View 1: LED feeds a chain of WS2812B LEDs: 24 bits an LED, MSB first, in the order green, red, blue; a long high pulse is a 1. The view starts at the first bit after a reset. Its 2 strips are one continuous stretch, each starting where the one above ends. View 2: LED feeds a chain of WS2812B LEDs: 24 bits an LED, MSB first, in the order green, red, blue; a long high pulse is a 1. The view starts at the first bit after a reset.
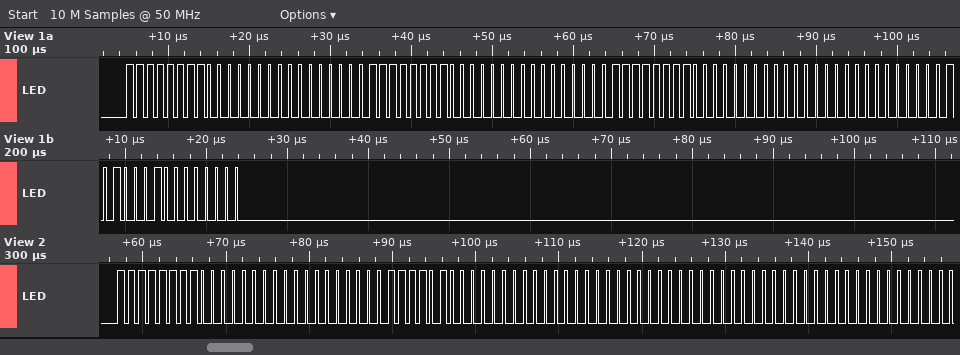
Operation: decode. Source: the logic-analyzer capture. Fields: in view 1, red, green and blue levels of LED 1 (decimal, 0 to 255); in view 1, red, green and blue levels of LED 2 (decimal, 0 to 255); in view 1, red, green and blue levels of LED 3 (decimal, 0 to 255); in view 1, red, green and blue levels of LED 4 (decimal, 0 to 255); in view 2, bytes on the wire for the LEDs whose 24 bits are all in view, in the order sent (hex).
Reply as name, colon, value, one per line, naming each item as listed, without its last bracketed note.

in view 1, red, green and blue levels of LED 1: 0, 255, 0
in view 1, red, green and blue levels of LED 2: 0, 255, 0
in view 1, red, green and blue levels of LED 3: 0, 255, 0
in view 1, red, green and blue levels of LED 4: 81, 0, 0
in view 2, bytes on the wire for the LEDs whose 24 bits are all in view, in the order sent: FF 00 00 3D 00 00 00 00 00
